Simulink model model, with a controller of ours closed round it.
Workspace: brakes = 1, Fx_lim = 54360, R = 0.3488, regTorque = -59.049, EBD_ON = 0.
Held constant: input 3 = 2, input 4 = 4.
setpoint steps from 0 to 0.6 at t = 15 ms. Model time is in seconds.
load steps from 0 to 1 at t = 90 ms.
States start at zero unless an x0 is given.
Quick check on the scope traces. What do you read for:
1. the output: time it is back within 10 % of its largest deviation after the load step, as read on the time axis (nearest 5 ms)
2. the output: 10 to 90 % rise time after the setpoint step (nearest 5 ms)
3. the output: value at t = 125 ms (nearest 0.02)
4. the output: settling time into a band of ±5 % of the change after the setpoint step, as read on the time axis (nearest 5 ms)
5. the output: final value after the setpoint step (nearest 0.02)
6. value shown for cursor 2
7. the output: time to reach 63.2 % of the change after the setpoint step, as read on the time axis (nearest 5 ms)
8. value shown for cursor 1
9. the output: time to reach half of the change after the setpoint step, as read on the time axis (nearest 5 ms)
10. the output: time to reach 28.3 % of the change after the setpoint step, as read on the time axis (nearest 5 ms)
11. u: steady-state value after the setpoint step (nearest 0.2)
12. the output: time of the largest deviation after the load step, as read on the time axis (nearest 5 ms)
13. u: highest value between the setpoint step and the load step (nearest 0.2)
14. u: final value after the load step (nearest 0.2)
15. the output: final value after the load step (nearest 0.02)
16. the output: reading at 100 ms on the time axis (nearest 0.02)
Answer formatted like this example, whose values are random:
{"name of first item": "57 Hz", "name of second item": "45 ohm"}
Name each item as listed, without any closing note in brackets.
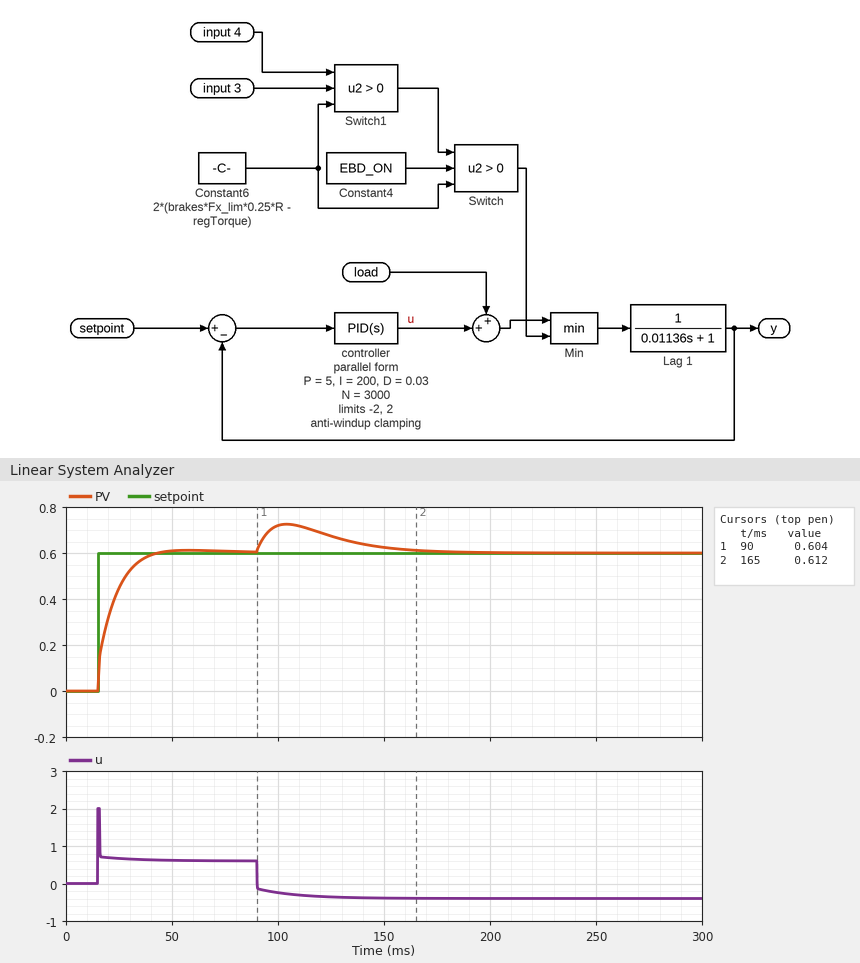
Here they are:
{"the output: time it is back within 10 % of its largest deviation after the load step, as read on the time axis": "165 ms", "the output: 10 to 90 % rise time after the setpoint step": "15 ms", "the output: value at t = 125 ms": "0.68", "the output: settling time into a band of ±5 % of the change after the setpoint step, as read on the time axis": "35 ms", "the output: final value after the setpoint step": "0.60", "value shown for cursor 2": "0.612", "the output: time to reach 63.2 % of the change after the setpoint step, as read on the time axis": "20 ms", "value shown for cursor 1": "0.604", "the output: time to reach half of the change after the setpoint step, as read on the time axis": "20 ms", "the output: time to reach 28.3 % of the change after the setpoint step, as read on the time axis": "15 ms", "u: steady-state value after the setpoint step": "0.6", "the output: time of the largest deviation after the load step, as read on the time axis": "105 ms", "u: highest value between the setpoint step and the load step": "2.0", "u: final value after the load step": "-0.4", "the output: final value after the load step": "0.60", "the output: reading at 100 ms on the time axis": "0.72"}
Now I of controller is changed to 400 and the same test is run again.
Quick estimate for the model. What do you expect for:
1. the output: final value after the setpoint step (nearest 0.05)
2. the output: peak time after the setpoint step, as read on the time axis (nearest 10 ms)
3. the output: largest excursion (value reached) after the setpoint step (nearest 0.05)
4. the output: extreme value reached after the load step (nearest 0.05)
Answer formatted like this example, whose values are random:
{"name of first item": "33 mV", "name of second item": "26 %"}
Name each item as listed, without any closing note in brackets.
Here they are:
{"the output: final value after the setpoint step": "0.60", "the output: peak time after the setpoint step, as read on the time axis": "40 ms", "the output: largest excursion (value reached) after the setpoint step": "0.65", "the output: extreme value reached after the load step": "0.70"}
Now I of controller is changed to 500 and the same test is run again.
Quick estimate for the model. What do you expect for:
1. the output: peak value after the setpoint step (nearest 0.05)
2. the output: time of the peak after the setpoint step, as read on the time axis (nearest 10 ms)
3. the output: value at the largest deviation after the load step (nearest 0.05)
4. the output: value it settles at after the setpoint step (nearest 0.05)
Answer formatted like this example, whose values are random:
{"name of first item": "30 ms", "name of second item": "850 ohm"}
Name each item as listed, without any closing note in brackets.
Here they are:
{"the output: peak value after the setpoint step": "0.65", "the output: time of the peak after the setpoint step, as read on the time axis": "40 ms", "the output: value at the largest deviation after the load step": "0.70", "the output: value it settles at after the setpoint step": "0.60"}
